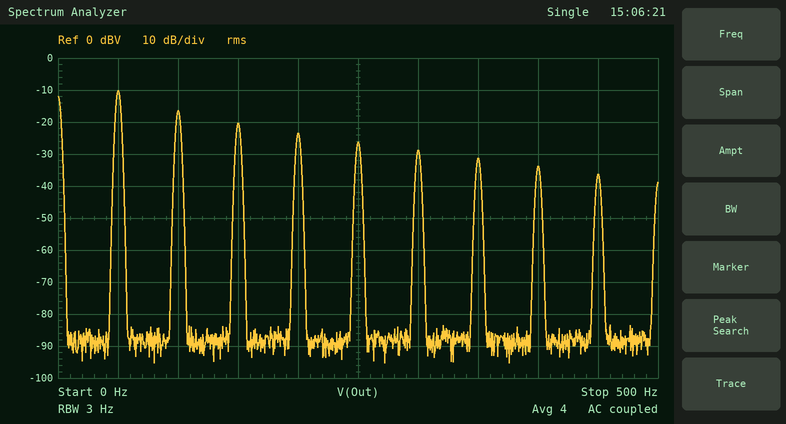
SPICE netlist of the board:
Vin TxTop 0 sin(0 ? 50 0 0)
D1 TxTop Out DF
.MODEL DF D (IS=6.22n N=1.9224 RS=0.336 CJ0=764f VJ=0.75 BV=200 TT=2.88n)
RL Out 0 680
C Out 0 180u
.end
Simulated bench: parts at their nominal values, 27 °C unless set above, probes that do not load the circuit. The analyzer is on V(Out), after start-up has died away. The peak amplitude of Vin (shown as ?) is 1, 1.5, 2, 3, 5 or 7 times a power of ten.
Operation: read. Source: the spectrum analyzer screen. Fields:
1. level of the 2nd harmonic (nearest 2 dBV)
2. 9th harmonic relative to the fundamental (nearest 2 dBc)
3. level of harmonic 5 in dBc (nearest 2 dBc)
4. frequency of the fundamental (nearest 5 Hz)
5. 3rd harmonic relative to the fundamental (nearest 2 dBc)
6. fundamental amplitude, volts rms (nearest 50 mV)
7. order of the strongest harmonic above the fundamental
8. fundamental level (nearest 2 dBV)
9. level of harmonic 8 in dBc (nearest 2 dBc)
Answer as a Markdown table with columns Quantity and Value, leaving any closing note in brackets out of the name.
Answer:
| Quantity | Value |
|---|---|
| level of the 2nd harmonic | -16 dBV |
| 9th harmonic relative to the fundamental | -26 dBc |
| level of harmonic 5 in dBc | -16 dBc |
| frequency of the fundamental | 50 Hz |
| 3rd harmonic relative to the fundamental | -10 dBc |
| fundamental amplitude, volts rms | 300 mV |
| order of the strongest harmonic above the fundamental | 2 |
| fundamental level | -10 dBV |
| level of harmonic 8 in dBc | -24 dBc |
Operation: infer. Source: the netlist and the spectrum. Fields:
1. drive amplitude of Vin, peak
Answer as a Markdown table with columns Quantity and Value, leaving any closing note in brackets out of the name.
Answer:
| Quantity | Value |
|---|---|
| drive amplitude of Vin, peak | 10 V |
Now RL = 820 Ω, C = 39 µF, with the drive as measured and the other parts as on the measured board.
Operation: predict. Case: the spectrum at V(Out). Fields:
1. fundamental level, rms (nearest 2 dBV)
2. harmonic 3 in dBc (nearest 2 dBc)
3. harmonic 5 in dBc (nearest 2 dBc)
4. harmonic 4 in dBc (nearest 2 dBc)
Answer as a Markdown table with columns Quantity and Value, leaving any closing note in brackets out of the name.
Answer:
| Quantity | Value |
|---|---|
| fundamental level, rms | 0 dBV |
| harmonic 3 in dBc | -12 dBc |
| harmonic 5 in dBc | -20 dBc |
| harmonic 4 in dBc | -16 dBc |
